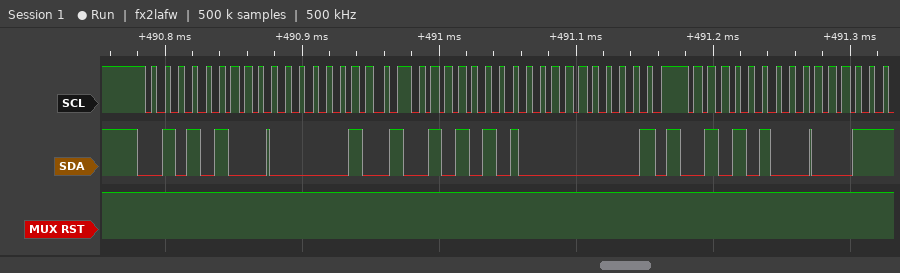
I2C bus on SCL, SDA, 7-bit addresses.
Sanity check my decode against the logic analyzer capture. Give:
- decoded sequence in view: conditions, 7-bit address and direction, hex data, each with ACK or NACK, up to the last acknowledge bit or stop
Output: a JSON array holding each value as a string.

["start, address 2A write ACK, 02 ACK, repeated start, address 2A read ACK, 00 NACK, stop, start, address 2A write ACK"]
